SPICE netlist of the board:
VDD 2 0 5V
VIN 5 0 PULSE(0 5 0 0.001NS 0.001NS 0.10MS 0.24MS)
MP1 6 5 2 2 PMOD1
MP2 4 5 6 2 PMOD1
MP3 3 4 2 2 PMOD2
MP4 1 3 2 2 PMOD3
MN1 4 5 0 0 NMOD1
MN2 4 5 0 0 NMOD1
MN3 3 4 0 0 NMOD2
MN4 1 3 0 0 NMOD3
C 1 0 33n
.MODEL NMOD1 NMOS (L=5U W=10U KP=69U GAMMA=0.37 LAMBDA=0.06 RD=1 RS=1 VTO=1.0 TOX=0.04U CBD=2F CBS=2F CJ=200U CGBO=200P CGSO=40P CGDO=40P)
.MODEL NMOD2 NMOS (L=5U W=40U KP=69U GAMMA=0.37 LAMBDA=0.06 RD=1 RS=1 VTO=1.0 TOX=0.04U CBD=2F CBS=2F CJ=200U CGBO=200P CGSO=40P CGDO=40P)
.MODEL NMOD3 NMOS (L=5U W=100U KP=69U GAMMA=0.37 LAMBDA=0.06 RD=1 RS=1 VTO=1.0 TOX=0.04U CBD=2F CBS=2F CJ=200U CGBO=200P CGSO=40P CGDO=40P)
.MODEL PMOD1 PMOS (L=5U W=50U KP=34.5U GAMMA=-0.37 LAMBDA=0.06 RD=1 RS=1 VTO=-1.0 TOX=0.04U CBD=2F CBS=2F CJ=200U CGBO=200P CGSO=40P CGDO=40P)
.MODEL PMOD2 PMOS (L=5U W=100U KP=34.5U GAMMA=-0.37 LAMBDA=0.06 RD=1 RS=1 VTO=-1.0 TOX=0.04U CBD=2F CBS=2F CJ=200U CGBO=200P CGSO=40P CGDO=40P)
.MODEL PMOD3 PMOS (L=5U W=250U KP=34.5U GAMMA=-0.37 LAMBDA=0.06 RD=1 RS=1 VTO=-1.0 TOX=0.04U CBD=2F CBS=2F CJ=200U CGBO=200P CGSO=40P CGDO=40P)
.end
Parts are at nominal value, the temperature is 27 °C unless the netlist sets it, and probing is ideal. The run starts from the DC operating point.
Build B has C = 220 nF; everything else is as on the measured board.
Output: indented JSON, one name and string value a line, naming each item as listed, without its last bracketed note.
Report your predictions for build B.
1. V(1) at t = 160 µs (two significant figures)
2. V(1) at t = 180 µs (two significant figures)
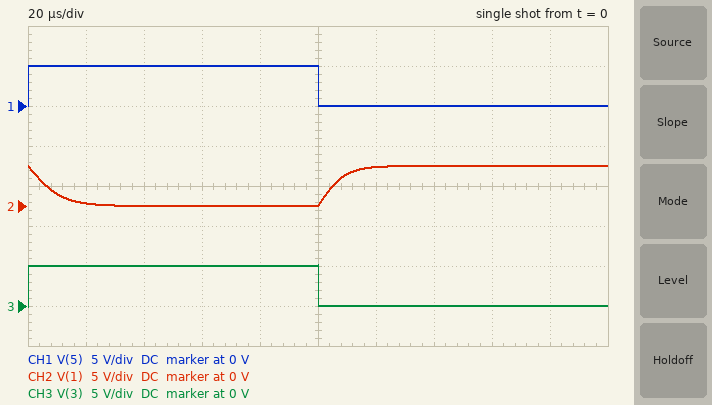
{
  "V(1) at t = 160 µs": "4.0 V",
  "V(1) at t = 180 µs": "4.5 V"
}
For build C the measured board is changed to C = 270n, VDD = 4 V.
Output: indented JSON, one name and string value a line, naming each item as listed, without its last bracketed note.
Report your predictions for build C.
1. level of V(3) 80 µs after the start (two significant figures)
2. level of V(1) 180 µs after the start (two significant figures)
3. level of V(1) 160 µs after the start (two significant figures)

{
  "level of V(3) 80 µs after the start": "4.0 V",
  "level of V(1) 180 µs after the start": "3.3 V",
  "level of V(1) 160 µs after the start": "3.0 V"
}
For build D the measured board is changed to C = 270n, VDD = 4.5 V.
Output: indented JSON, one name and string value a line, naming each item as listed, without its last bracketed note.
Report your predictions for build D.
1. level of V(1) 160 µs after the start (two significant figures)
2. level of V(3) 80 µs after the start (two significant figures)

{
  "level of V(1) 160 µs after the start": "3.4 V",
  "level of V(3) 80 µs after the start": "4.5 V"
}
